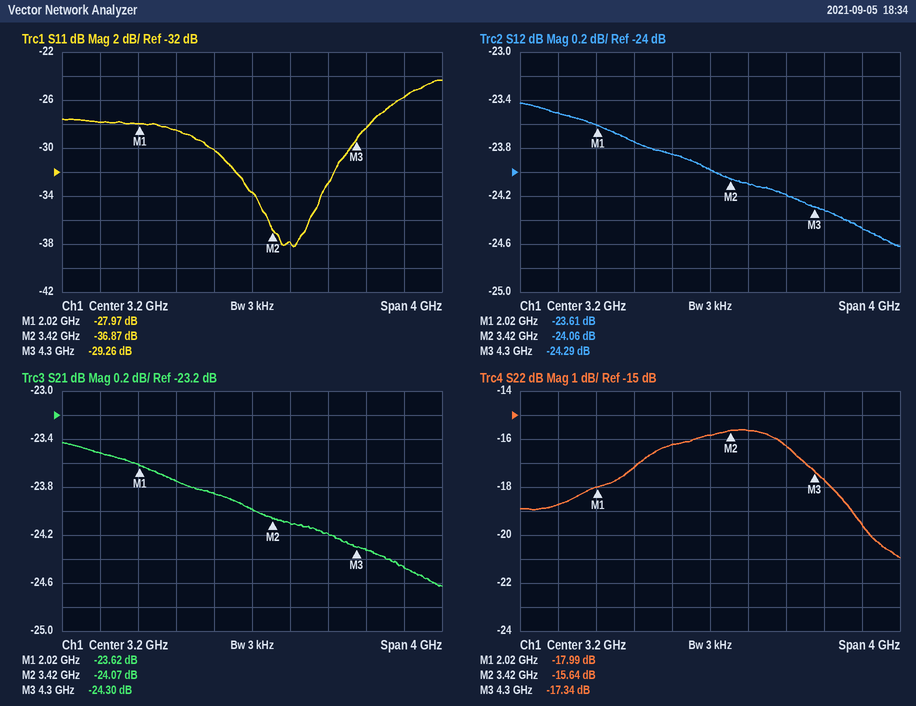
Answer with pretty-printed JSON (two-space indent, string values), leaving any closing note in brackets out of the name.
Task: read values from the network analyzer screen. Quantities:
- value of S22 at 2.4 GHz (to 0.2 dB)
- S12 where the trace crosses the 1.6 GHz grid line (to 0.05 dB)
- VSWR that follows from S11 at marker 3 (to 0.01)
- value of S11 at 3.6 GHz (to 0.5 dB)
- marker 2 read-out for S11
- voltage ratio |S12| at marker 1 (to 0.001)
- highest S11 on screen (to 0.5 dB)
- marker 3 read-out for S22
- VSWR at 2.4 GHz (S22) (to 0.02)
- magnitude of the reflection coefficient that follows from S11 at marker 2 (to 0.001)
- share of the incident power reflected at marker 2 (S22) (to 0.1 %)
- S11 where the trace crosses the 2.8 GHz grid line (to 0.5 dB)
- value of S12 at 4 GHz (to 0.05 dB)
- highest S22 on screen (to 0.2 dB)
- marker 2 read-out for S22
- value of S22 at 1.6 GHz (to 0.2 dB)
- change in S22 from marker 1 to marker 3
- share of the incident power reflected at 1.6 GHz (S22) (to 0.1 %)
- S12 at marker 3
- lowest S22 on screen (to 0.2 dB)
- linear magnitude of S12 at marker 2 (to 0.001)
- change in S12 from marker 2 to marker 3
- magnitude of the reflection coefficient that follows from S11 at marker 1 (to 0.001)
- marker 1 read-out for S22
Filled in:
{
  "value of S22 at 2.4 GHz": "-17.2 dB",
  "S12 where the trace crosses the 1.6 GHz grid line": "-23.50 dB",
  "VSWR that follows from S11 at marker 3": "1.07",
  "value of S11 at 3.6 GHz": "-38.0 dB",
  "marker 2 read-out for S11": "-36.87 dB",
  "voltage ratio |S12| at marker 1": "0.066",
  "highest S11 on screen": "-24.5 dB",
  "marker 3 read-out for S22": "-17.34 dB",
  "VSWR at 2.4 GHz (S22)": "1.32",
  "magnitude of the reflection coefficient that follows from S11 at marker 2": "0.014",
  "share of the incident power reflected at marker 2 (S22)": "2.7 %",
  "S11 where the trace crosses the 2.8 GHz grid line": "-30.0 dB",
  "value of S12 at 4 GHz": "-24.20 dB",
  "highest S22 on screen": "-15.6 dB",
  "marker 2 read-out for S22": "-15.64 dB",
  "value of S22 at 1.6 GHz": "-18.8 dB",
  "change in S22 from marker 1 to marker 3": "0.65 dB",
  "share of the incident power reflected at 1.6 GHz (S22)": "1.3 %",
  "S12 at marker 3": "-24.29 dB",
  "lowest S22 on screen": "-21.0 dB",
  "linear magnitude of S12 at marker 2": "0.063",
  "change in S12 from marker 2 to marker 3": "-0.23 dB",
  "magnitude of the reflection coefficient that follows from S11 at marker 1": "0.040",
  "marker 1 read-out for S22": "-17.99 dB"
}
